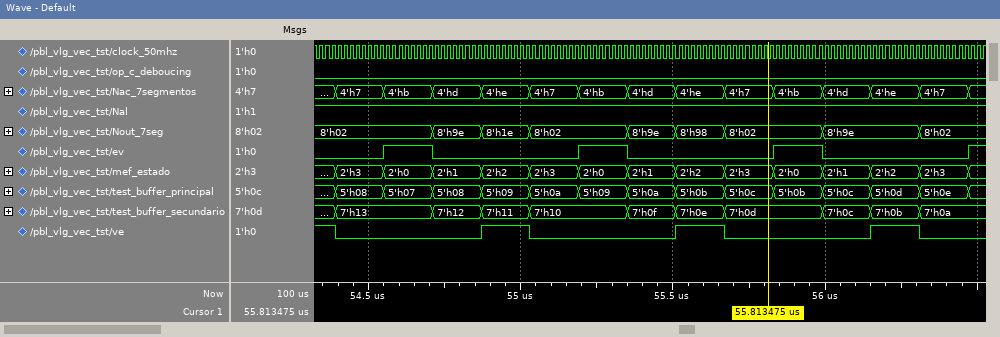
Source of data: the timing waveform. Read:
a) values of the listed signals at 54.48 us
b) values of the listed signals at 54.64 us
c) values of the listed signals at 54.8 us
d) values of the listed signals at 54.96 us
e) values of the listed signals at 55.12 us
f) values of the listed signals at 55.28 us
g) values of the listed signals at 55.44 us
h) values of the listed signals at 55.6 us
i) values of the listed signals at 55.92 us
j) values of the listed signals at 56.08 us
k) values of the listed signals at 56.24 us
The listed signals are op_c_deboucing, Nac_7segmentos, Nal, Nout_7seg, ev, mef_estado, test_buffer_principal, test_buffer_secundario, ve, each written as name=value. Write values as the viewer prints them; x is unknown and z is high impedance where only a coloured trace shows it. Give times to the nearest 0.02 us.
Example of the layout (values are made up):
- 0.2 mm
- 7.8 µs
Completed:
- op_c_deboucing=0, Nac_7segmentos=4'h7, Nal=1, Nout_7seg=8'h02, ev=0, mef_estado=2'h3, test_buffer_principal=5'h08, test_buffer_secundario=7'h13, ve=0
- op_c_deboucing=0, Nac_7segmentos=4'hb, Nal=1, Nout_7seg=8'h02, ev=1, mef_estado=2'h0, test_buffer_principal=5'h07, test_buffer_secundario=7'h13, ve=0
- op_c_deboucing=0, Nac_7segmentos=4'hd, Nal=1, Nout_7seg=8'h9e, ev=0, mef_estado=2'h1, test_buffer_principal=5'h08, test_buffer_secundario=7'h12, ve=0
- op_c_deboucing=0, Nac_7segmentos=4'he, Nal=1, Nout_7seg=8'h1e, ev=0, mef_estado=2'h2, test_buffer_principal=5'h09, test_buffer_secundario=7'h11, ve=1
- op_c_deboucing=0, Nac_7segmentos=4'h7, Nal=1, Nout_7seg=8'h02, ev=0, mef_estado=2'h3, test_buffer_principal=5'h0a, test_buffer_secundario=7'h10, ve=0
- op_c_deboucing=0, Nac_7segmentos=4'hb, Nal=1, Nout_7seg=8'h02, ev=1, mef_estado=2'h0, test_buffer_principal=5'h09, test_buffer_secundario=7'h10, ve=0
- op_c_deboucing=0, Nac_7segmentos=4'hd, Nal=1, Nout_7seg=8'h9e, ev=0, mef_estado=2'h1, test_buffer_principal=5'h0a, test_buffer_secundario=7'h0f, ve=0
- op_c_deboucing=0, Nac_7segmentos=4'he, Nal=1, Nout_7seg=8'h98, ev=0, mef_estado=2'h2, test_buffer_principal=5'h0b, test_buffer_secundario=7'h0e, ve=1
- op_c_deboucing=0, Nac_7segmentos=4'hb, Nal=1, Nout_7seg=8'h02, ev=1, mef_estado=2'h0, test_buffer_principal=5'h0b, test_buffer_secundario=7'h0d, ve=0
- op_c_deboucing=0, Nac_7segmentos=4'hd, Nal=1, Nout_7seg=8'h9e, ev=0, mef_estado=2'h1, test_buffer_principal=5'h0c, test_buffer_secundario=7'h0c, ve=0
- op_c_deboucing=0, Nac_7segmentos=4'he, Nal=1, Nout_7seg=8'h9e, ev=0, mef_estado=2'h2, test_buffer_principal=5'h0d, test_buffer_secundario=7'h0b, ve=1
